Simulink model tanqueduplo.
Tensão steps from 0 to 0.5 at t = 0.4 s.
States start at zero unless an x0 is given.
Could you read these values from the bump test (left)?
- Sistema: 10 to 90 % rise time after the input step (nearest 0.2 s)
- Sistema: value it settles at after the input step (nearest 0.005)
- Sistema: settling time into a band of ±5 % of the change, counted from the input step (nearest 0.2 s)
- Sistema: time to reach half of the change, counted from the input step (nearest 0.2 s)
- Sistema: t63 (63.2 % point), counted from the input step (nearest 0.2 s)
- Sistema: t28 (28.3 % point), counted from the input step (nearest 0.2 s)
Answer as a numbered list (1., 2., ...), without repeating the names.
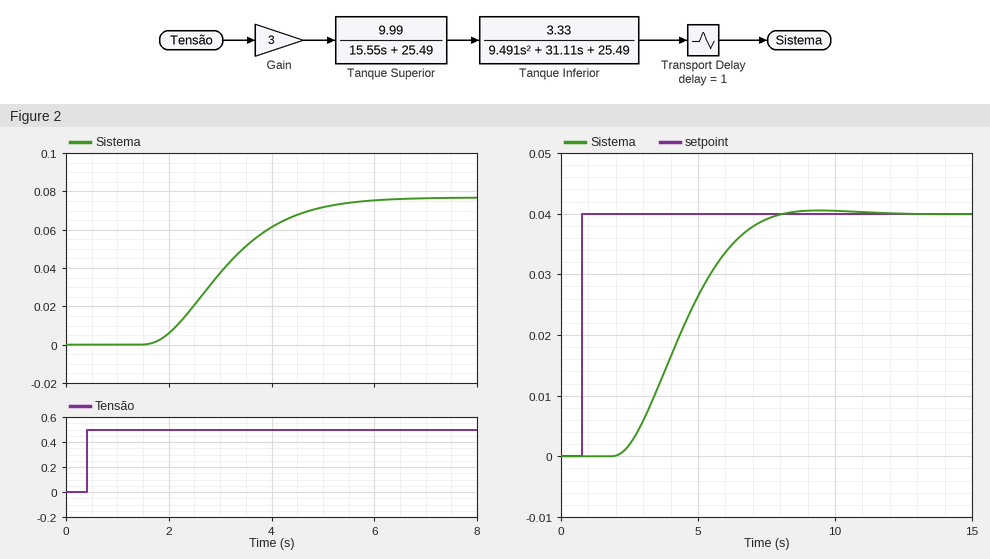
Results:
1. 2.6 s
2. 0.075
3. 4.8 s
4. 2.6 s
5. 3.0 s
6. 2.2 s
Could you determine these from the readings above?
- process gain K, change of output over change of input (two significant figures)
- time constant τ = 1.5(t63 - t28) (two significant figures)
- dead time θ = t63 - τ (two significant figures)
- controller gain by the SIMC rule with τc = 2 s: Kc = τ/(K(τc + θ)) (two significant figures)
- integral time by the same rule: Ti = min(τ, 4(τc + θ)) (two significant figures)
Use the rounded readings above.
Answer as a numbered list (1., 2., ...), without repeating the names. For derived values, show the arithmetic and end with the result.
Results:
1. (0.075 - 0) / 0.5 = 0.15
2. 1.5 × (3 - 2.2) = 1.2 s
3. 3 - 1.2 = 1.8 s
4. 1.2 / (0.15 × (2 + 1.8)) = 2.1
5. min(1.2, 4 × (2 + 1.8)) = 1.2 s
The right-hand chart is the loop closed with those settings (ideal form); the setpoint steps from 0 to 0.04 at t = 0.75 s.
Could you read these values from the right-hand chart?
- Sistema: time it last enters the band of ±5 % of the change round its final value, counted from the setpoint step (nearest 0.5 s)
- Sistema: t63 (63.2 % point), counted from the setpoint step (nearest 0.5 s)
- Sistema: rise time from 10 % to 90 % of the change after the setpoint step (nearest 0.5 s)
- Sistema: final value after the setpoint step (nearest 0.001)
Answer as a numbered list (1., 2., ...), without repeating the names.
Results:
1. 6.5 s
2. 4.0 s
3. 3.5 s
4. 0.040
